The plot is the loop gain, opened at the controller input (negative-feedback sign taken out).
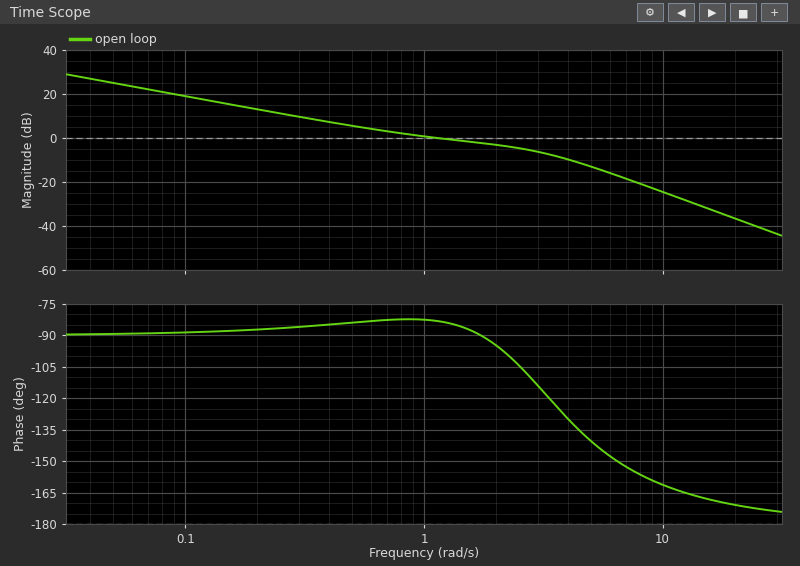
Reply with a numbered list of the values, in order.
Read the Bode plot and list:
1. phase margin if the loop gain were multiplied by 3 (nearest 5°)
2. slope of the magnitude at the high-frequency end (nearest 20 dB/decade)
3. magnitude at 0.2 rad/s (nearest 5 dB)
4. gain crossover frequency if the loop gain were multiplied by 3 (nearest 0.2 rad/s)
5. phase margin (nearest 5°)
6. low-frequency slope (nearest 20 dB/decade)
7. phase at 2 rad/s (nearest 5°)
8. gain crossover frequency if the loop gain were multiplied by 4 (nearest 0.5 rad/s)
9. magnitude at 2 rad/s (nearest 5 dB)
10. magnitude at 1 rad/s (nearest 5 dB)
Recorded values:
1. 50°
2. -40 dB/decade
3. 15 dB
4. 4.0 rad/s
5. 95°
6. -20 dB/decade
7. -95°
8. 4.5 rad/s
9. -5 dB
10. 0 dB
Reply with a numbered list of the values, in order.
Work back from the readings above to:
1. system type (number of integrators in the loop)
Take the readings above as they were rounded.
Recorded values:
1. 1
